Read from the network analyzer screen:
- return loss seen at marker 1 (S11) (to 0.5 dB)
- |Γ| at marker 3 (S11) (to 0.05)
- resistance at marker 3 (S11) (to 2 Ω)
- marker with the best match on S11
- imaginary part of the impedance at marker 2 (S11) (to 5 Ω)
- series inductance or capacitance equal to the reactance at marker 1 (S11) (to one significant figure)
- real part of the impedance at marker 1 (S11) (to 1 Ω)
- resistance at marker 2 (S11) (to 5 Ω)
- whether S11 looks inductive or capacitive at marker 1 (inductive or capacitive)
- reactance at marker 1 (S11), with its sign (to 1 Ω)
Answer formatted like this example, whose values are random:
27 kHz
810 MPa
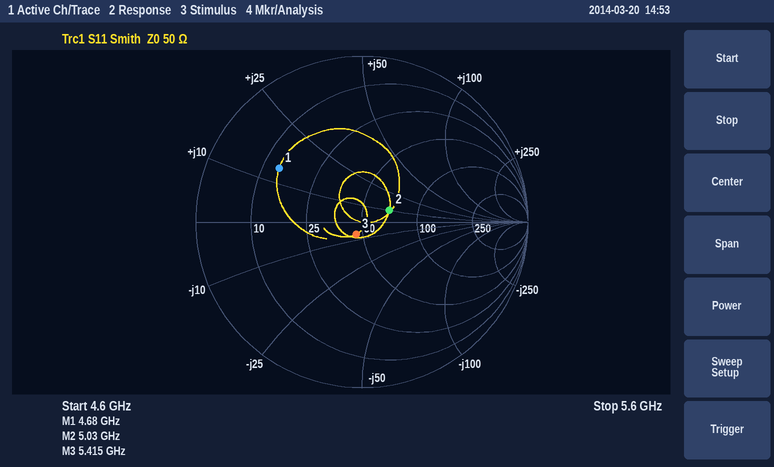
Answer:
4.5 dB
0.10
46 Ω
marker 3
+10 Ω
500 pH
14 Ω
70 Ω
inductive
+14 Ω
